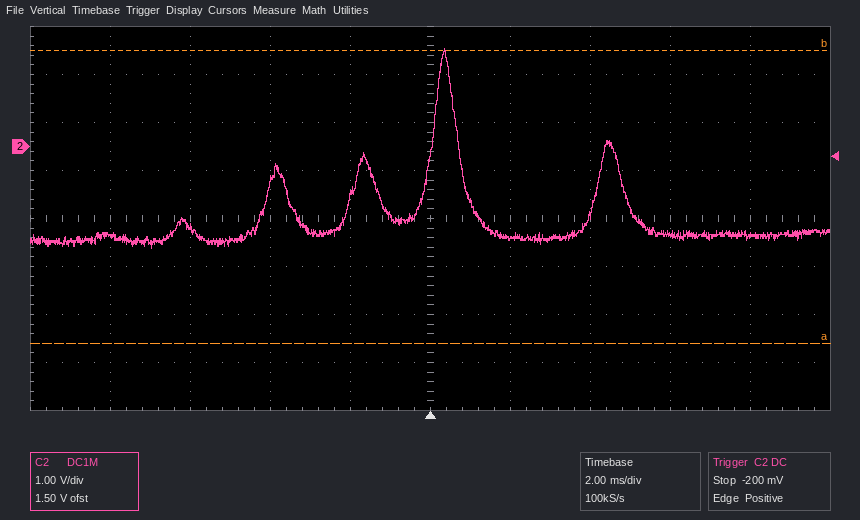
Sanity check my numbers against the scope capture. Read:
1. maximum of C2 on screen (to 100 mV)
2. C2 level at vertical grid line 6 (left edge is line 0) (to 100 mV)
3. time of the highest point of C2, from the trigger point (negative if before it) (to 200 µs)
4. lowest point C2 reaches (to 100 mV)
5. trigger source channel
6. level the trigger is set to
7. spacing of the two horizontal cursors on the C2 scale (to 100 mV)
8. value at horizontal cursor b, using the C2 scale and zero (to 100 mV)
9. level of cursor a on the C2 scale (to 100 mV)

2.0 V
-1.9 V
+400 µs
-2.1 V
C2
-200 mV
6.1 V
2.0 V
-4.1 V
